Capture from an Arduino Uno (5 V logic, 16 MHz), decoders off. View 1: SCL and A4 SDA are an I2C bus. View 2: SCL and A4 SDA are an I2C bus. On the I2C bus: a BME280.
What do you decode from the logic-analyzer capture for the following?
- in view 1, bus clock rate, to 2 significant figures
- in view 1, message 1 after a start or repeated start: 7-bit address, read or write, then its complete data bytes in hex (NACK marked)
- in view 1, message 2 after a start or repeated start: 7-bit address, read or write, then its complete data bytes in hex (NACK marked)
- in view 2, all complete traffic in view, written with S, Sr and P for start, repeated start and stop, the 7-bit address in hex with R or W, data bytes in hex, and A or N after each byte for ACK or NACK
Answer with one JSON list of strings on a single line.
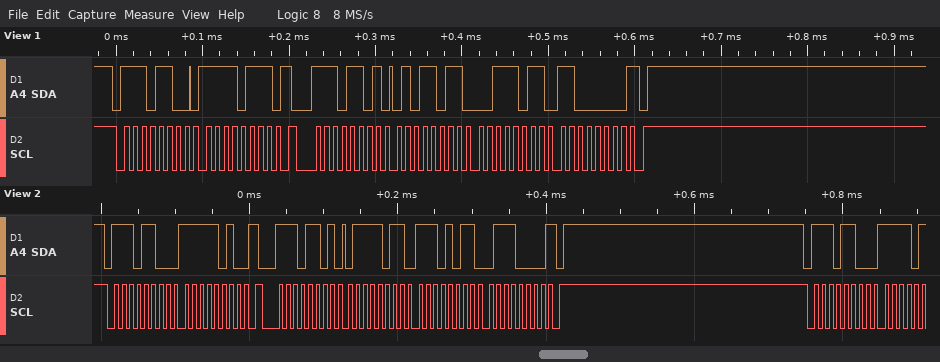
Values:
["100 kHz", "0x76 write: F7", "0x76 read: 5B 3B C0 NACK", "S 76W A FA A Sr 76R A 7B A EB A 70 N P S 76W A"]
